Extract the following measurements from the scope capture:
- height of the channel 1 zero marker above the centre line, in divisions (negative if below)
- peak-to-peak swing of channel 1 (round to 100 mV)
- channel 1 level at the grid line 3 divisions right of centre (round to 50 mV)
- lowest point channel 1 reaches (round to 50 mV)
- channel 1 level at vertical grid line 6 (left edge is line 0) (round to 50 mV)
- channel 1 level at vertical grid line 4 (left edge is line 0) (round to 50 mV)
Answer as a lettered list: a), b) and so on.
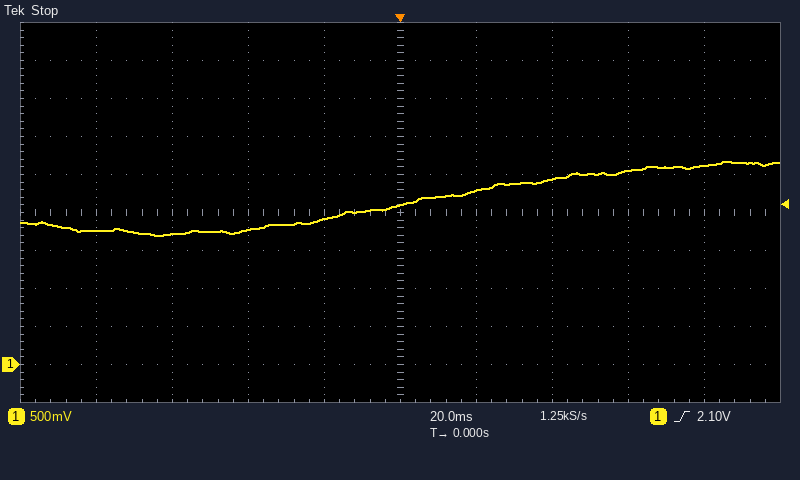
a) -4.0 div
b) 1.00 V
c) 2.55 V
d) 1.70 V
e) 2.30 V
f) 1.90 V
